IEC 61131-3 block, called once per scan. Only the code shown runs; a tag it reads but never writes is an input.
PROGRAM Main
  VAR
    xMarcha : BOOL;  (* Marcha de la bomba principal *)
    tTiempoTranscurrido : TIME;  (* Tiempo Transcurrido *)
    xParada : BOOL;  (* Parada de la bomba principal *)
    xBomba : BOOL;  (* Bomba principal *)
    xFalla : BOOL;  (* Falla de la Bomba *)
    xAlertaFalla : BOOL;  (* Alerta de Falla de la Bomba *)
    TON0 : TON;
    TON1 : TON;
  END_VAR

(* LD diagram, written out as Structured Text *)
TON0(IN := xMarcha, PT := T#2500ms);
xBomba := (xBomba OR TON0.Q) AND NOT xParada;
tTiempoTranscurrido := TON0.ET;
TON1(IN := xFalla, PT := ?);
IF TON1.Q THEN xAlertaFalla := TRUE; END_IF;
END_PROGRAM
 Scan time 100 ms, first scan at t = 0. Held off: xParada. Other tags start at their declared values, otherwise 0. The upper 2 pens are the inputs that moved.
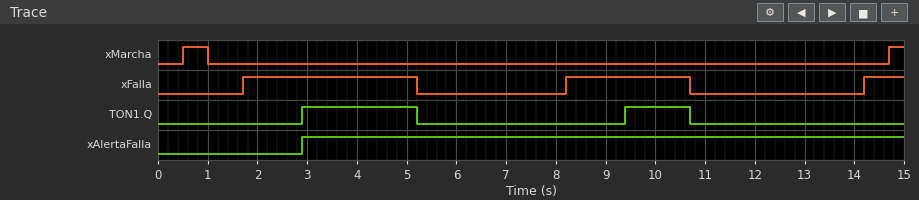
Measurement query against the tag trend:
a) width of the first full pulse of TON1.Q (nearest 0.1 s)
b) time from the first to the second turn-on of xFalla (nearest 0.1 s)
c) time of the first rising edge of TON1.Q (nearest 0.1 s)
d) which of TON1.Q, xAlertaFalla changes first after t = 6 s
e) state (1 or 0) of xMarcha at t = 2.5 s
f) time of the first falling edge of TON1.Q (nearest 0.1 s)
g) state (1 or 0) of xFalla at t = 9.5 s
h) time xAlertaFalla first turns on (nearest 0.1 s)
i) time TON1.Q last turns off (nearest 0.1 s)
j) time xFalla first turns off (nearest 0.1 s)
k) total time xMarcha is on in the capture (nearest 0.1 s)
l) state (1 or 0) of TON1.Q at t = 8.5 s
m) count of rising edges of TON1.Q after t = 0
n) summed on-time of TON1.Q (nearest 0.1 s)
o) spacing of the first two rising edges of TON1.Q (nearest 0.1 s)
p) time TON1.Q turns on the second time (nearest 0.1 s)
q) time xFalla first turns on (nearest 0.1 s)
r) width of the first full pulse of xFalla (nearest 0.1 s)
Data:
2.3 s
6.5 s
2.9 s
TON1.Q
0
5.2 s
1
2.9 s
10.7 s
5.2 s
0.8 s
0
2
3.6 s
6.5 s
9.4 s
1.7 s
3.5 s
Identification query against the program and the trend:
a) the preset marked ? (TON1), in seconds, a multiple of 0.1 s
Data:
1.2 s
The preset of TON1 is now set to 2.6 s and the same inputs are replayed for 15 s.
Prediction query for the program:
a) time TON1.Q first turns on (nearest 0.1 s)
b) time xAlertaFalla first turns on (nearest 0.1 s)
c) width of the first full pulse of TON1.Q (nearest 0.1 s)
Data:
4.3 s
4.3 s
0.9 s
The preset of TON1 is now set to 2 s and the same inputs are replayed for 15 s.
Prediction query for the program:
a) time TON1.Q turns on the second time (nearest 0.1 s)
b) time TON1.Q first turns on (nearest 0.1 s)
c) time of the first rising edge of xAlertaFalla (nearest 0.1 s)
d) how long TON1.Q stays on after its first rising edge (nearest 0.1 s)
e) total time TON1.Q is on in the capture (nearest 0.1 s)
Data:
10.2 s
3.7 s
3.7 s
1.5 s
2.0 s
